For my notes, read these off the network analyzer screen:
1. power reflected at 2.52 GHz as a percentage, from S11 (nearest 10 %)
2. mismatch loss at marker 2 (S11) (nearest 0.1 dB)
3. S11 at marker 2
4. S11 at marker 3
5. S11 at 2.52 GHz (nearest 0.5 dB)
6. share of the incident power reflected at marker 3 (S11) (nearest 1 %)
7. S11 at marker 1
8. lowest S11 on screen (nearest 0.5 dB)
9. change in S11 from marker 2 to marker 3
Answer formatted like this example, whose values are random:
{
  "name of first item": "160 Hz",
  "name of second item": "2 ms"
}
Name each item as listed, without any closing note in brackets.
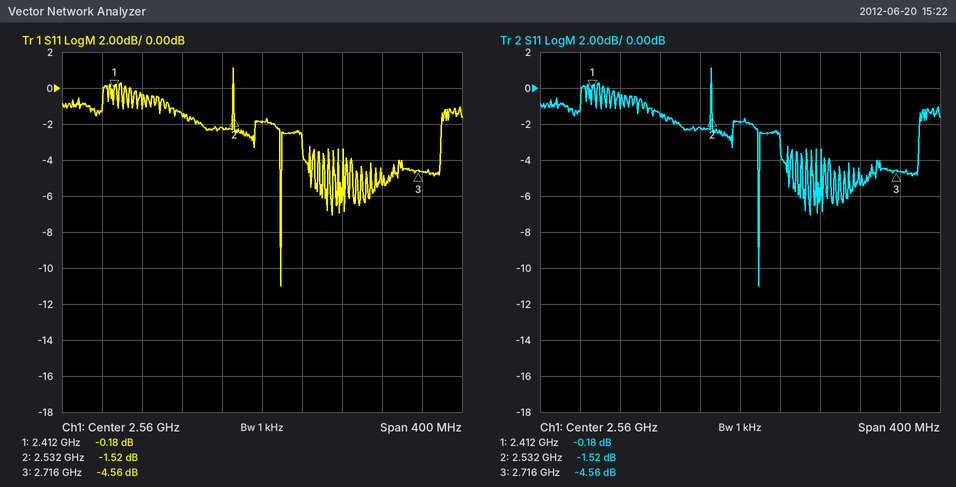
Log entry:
{
  "power reflected at 2.52 GHz as a percentage, from S11": "60 %",
  "mismatch loss at marker 2 (S11)": "5.3 dB",
  "S11 at marker 2": "-1.52 dB",
  "S11 at marker 3": "-4.56 dB",
  "S11 at 2.52 GHz": "-2.0 dB",
  "share of the incident power reflected at marker 3 (S11)": "35 %",
  "S11 at marker 1": "-0.18 dB",
  "lowest S11 on screen": "-11.0 dB",
  "change in S11 from marker 2 to marker 3": "-3.04 dB"
}
